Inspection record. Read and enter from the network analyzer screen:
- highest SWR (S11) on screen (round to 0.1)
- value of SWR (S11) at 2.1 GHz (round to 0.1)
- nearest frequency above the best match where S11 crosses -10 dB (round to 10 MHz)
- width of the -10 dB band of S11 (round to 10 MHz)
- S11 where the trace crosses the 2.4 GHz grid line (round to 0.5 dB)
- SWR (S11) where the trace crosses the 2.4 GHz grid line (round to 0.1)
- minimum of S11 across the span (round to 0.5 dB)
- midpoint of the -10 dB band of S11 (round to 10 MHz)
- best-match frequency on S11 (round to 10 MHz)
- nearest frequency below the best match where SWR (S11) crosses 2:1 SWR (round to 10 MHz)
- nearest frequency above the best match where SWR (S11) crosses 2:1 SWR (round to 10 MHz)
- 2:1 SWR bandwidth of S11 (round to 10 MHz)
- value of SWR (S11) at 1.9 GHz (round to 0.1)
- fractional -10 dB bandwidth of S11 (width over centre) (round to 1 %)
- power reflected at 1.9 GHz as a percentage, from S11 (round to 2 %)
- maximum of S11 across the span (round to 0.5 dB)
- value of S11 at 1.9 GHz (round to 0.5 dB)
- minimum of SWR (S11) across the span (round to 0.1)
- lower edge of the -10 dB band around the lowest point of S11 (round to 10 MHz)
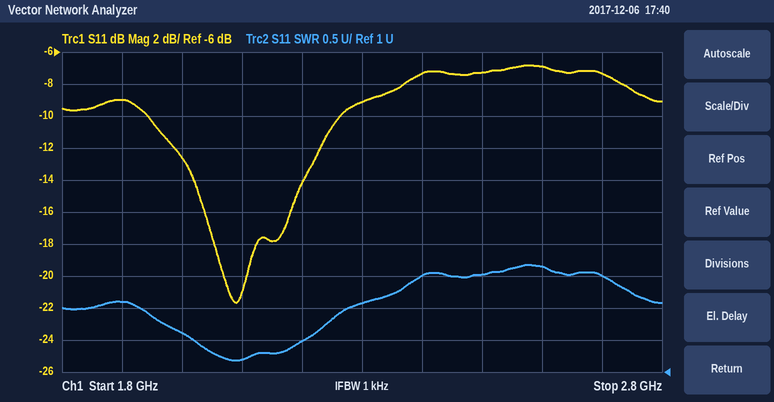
2.7
1.2
2.26 GHz
320 MHz
-7.5 dB
2.5
-21.5 dB
2.10 GHz
2.09 GHz
1.93 GHz
2.28 GHz
350 MHz
2.1
15 %
12 %
-7.0 dB
-9.0 dB
1.2
1.94 GHz
